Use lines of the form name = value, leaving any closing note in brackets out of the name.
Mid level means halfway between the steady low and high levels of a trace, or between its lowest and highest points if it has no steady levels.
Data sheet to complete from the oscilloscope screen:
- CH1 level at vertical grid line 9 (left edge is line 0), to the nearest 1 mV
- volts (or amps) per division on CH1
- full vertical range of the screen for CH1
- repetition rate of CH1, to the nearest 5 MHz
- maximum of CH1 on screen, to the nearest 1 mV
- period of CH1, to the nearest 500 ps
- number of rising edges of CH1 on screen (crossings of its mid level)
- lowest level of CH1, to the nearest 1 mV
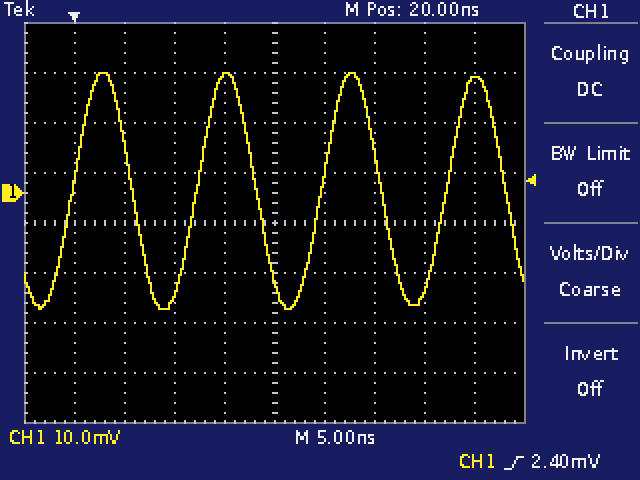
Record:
CH1 level at vertical grid line 9 (left edge is line 0), to the nearest 1 mV = 23 mV
volts (or amps) per division on CH1 = 10 mV
full vertical range of the screen for CH1 = 80 mV
repetition rate of CH1, to the nearest 5 MHz = 80 MHz
maximum of CH1 on screen, to the nearest 1 mV = 24 mV
period of CH1, to the nearest 500 ps = 12.5 ns
number of rising edges of CH1 on screen = 4
lowest level of CH1, to the nearest 1 mV = -23 mV
